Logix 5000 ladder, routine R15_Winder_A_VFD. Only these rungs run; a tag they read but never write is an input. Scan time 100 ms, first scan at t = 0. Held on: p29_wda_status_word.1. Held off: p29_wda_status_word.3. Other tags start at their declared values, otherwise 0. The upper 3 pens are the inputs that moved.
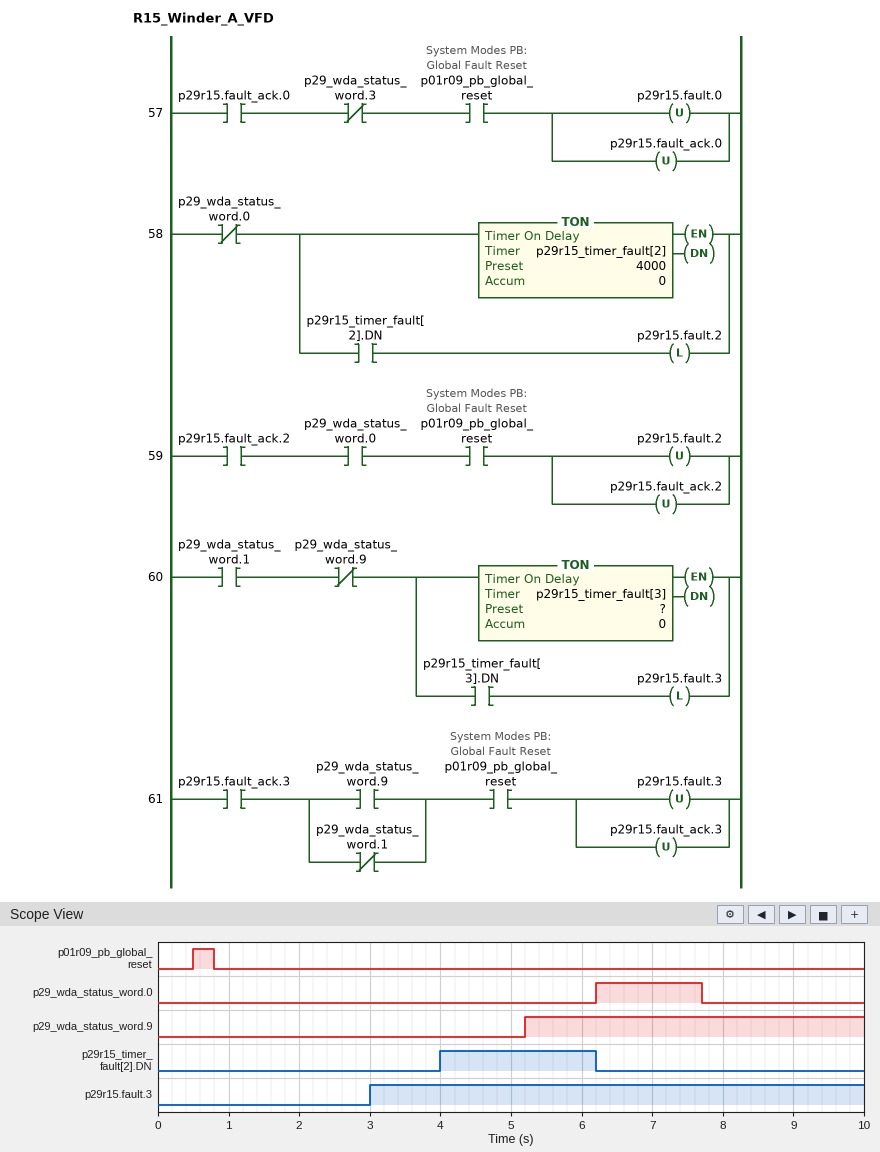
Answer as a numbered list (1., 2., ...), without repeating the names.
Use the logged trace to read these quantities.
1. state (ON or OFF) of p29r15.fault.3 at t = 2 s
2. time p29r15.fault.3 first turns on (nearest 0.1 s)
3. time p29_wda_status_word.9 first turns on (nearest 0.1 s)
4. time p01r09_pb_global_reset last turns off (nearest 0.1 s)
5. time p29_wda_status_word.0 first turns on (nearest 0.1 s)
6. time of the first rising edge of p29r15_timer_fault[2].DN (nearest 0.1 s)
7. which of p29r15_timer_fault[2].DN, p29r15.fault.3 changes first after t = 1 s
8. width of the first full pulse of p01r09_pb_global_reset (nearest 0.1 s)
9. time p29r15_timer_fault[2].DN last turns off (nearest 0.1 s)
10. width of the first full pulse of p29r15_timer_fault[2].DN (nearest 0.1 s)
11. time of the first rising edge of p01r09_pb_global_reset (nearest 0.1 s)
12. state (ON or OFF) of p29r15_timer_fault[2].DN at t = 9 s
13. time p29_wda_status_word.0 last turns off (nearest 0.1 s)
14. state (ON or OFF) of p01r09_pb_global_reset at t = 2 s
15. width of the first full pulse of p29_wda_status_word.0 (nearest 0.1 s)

1. OFF
2. 3.0 s
3. 5.2 s
4. 0.8 s
5. 6.2 s
6. 4.0 s
7. p29r15.fault.3
8. 0.3 s
9. 6.2 s
10. 2.2 s
11. 0.5 s
12. OFF
13. 7.7 s
14. OFF
15. 1.5 s
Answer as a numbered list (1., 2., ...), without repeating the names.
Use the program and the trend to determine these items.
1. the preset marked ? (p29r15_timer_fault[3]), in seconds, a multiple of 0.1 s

1. 3.0 s
